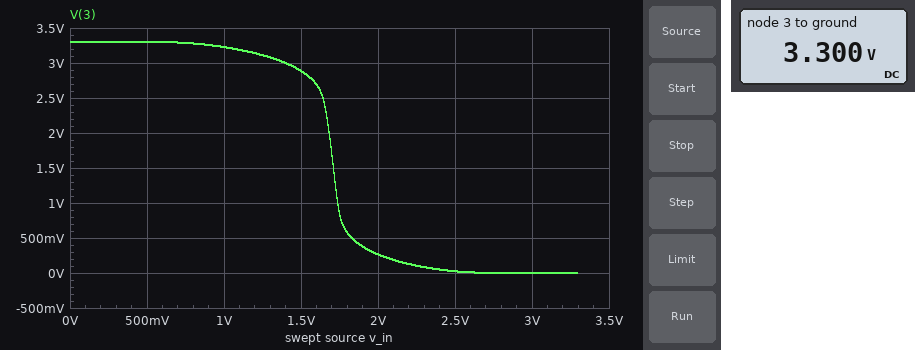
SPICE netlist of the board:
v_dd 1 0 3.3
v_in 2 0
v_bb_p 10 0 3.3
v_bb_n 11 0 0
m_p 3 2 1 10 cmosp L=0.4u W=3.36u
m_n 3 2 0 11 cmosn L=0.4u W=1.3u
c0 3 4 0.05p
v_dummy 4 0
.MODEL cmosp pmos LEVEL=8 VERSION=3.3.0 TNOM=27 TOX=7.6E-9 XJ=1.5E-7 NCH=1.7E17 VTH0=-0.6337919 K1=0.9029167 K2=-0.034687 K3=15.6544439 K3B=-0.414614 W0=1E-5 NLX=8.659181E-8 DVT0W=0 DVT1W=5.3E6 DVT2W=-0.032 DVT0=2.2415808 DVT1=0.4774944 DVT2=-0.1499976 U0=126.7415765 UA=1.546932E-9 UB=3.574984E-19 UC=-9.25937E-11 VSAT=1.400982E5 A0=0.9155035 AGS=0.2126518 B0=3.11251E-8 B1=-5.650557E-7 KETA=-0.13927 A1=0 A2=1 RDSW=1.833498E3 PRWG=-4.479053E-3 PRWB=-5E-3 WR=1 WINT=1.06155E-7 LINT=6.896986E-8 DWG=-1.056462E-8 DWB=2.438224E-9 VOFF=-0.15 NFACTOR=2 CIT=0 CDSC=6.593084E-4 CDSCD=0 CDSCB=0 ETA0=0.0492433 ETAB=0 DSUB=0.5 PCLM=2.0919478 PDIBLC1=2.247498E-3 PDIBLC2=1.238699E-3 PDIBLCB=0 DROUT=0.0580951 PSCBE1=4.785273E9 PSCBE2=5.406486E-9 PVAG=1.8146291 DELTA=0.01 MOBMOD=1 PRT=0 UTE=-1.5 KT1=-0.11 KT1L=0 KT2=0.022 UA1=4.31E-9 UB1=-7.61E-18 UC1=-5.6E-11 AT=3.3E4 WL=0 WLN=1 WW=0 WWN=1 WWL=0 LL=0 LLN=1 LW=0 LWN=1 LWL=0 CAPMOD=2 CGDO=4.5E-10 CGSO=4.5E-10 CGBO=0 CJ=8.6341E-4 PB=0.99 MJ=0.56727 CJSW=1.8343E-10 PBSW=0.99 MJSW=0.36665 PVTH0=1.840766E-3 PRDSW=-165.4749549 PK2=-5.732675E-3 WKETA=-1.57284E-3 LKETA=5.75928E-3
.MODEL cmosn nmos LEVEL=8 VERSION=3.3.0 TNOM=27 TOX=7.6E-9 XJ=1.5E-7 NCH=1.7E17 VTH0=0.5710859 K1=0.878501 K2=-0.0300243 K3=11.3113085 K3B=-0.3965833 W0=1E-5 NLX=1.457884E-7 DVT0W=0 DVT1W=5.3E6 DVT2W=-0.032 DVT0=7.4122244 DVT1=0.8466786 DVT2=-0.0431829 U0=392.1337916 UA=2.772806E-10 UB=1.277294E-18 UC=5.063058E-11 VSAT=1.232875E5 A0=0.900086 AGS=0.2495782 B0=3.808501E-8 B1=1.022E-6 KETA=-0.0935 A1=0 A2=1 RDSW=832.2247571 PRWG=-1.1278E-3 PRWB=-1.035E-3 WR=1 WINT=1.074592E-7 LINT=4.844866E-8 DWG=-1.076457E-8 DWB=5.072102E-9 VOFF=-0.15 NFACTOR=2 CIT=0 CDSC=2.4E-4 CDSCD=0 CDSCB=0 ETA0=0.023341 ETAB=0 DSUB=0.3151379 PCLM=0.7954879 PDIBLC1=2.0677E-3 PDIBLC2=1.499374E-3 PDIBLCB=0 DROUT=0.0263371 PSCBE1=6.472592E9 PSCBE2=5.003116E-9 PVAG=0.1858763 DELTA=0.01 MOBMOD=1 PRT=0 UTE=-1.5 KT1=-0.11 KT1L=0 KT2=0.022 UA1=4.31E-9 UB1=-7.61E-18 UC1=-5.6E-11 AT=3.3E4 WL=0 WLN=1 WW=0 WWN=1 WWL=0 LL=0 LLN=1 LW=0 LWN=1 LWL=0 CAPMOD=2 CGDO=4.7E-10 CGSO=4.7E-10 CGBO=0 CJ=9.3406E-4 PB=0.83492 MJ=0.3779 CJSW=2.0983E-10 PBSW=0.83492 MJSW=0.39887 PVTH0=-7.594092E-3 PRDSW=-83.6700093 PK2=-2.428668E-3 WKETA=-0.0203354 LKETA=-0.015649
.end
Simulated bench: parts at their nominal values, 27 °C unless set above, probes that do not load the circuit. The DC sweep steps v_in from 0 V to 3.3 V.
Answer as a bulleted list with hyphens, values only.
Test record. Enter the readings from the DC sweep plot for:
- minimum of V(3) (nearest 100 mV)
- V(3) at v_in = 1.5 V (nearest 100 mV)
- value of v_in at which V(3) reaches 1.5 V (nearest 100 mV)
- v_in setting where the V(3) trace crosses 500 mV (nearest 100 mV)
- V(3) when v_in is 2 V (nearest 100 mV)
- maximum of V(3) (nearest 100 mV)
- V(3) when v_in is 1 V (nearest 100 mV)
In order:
- 0 V
- 2.9 V
- 1.7 V
- 1.8 V
- 300 mV
- 3.3 V
- 3.2 V
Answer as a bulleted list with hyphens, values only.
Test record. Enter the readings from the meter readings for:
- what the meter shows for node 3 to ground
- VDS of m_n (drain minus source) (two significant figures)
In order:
- 3.300 V
- 3.3 V
